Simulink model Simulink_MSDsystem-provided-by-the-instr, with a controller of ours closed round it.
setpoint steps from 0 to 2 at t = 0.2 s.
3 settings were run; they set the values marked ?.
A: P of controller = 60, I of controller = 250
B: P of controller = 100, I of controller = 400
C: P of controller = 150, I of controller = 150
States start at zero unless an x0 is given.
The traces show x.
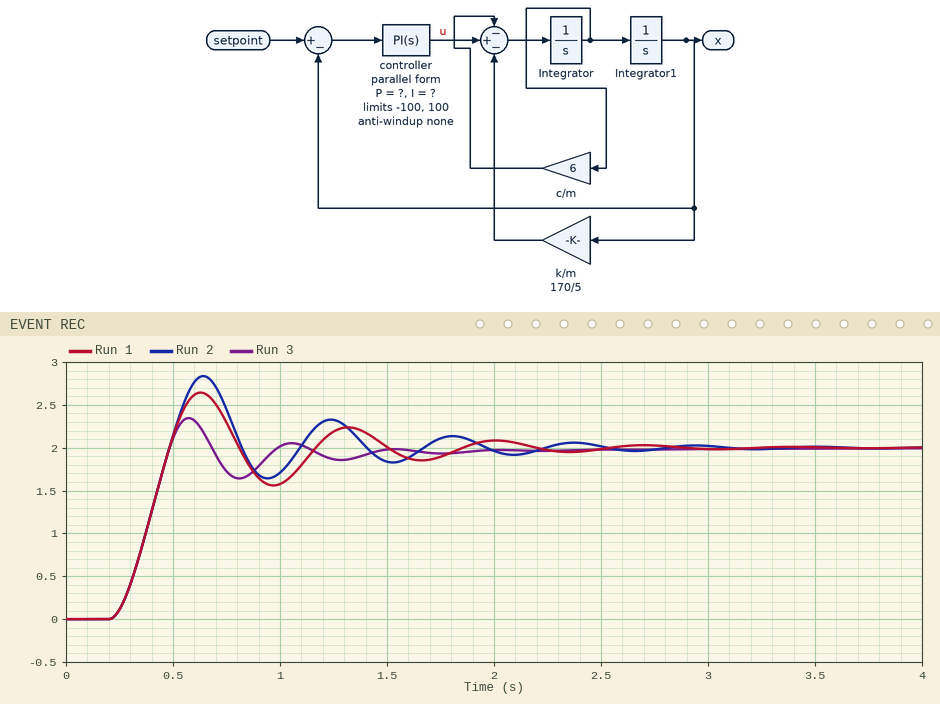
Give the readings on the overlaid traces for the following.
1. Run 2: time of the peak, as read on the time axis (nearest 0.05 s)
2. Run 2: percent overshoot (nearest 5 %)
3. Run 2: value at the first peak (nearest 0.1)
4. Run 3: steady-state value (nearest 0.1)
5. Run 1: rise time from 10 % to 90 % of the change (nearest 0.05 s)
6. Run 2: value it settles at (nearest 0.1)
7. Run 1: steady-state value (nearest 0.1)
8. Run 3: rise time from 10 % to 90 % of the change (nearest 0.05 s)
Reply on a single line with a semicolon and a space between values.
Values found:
0.65 s; 40 %; 2.8; 2.0; 0.20 s; 2.0; 2.0; 0.20 s
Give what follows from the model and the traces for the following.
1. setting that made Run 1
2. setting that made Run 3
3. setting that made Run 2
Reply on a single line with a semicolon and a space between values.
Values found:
A; C; B
